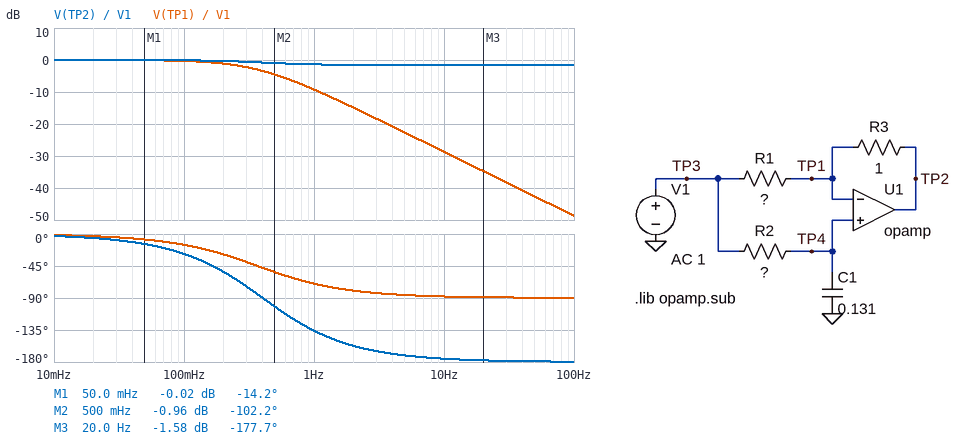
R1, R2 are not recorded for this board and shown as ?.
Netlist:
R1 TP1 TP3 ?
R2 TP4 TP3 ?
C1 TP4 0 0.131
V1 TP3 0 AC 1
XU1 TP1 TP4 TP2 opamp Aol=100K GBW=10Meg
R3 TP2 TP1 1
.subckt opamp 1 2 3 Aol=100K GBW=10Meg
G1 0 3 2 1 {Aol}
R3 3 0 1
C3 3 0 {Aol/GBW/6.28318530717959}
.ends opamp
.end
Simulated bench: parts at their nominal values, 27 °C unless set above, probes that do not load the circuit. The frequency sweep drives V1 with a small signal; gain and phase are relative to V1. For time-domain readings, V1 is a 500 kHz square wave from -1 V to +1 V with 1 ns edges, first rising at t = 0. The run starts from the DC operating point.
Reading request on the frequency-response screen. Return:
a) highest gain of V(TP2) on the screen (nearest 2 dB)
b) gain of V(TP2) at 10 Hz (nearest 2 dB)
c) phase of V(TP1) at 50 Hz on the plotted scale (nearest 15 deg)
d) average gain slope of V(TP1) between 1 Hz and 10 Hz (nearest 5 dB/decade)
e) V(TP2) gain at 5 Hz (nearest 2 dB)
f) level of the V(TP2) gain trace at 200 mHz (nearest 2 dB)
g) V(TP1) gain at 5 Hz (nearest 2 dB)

0 dB
-2 dB
-90 deg
-20 dB/decade
-2 dB
0 dB
-22 dB
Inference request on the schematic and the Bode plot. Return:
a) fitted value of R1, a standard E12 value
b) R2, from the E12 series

1.2 Ω
3.3 Ω
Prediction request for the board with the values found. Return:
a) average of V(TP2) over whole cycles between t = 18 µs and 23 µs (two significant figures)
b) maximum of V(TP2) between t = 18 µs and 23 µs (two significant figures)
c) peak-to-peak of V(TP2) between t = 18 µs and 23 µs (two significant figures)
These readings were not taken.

-1.8 V
-1.0 V
1.7 V
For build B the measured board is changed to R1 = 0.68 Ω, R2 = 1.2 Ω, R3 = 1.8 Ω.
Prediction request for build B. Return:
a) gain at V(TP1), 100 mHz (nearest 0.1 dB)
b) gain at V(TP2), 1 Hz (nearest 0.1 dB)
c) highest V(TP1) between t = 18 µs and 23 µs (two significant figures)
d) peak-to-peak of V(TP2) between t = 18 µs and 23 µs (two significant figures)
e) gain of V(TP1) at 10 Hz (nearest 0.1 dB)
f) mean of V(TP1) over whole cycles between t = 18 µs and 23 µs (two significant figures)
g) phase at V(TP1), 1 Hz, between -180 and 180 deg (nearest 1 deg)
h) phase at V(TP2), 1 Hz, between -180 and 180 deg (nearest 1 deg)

0 dB
6.0 dB
440 mV
5.3 V
-19.9 dB
-1.0 V
-45 deg
-114 deg
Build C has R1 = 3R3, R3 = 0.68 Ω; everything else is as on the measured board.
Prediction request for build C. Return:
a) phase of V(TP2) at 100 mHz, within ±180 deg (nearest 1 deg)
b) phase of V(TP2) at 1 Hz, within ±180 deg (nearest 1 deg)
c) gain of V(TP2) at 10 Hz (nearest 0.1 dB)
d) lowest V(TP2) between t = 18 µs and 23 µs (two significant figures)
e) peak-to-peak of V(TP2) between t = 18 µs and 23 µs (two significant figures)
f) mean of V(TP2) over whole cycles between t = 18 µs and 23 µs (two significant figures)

-18 deg
-99 deg
-13.6 dB
-1.4 V
410 mV
-1.2 V
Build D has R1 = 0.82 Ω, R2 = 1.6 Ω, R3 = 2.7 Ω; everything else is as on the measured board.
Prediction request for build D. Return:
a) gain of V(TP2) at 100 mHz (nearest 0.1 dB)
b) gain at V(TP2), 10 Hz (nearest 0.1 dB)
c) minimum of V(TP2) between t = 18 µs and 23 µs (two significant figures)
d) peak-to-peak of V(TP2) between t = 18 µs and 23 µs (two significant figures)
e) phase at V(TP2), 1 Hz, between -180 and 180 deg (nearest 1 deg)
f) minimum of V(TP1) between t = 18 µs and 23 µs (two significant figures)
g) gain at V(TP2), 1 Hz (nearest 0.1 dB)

0.7 dB
10.3 dB
-7.6 V
6.6 V
-130 deg
-2.5 V
8.6 dB
